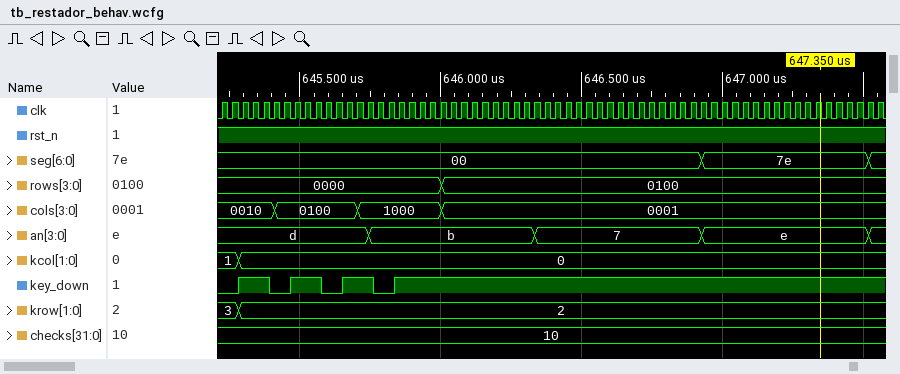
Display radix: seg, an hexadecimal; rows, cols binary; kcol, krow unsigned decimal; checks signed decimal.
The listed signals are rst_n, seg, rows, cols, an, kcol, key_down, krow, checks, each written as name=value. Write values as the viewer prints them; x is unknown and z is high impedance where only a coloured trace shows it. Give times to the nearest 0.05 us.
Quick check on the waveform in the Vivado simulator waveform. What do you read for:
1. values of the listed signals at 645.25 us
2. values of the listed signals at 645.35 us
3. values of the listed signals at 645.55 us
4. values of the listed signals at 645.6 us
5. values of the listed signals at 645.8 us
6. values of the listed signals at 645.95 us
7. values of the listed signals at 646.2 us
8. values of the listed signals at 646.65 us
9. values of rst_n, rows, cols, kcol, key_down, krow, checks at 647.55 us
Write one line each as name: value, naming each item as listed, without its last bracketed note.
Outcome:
values of the listed signals at 645.25 us: rst_n=1, seg=00, rows=0000, cols=0010, an=d, kcol=1, key_down=0, krow=3, checks=10
values of the listed signals at 645.35 us: rst_n=1, seg=00, rows=0000, cols=0010, an=d, kcol=0, key_down=1, krow=2, checks=10
values of the listed signals at 645.55 us: rst_n=1, seg=00, rows=0000, cols=0100, an=d, kcol=0, key_down=1, krow=2, checks=10
values of the listed signals at 645.6 us: rst_n=1, seg=00, rows=0000, cols=0100, an=d, kcol=0, key_down=0, krow=2, checks=10
values of the listed signals at 645.8 us: rst_n=1, seg=00, rows=0000, cols=1000, an=b, kcol=0, key_down=0, krow=2, checks=10
values of the listed signals at 645.95 us: rst_n=1, seg=00, rows=0000, cols=1000, an=b, kcol=0, key_down=1, krow=2, checks=10
values of the listed signals at 646.2 us: rst_n=1, seg=00, rows=0100, cols=0001, an=b, kcol=0, key_down=1, krow=2, checks=10
values of the listed signals at 646.65 us: rst_n=1, seg=00, rows=0100, cols=0001, an=7, kcol=0, key_down=1, krow=2, checks=10
values of rst_n, rows, cols, kcol, key_down, krow, checks at 647.55 us: rst_n=1, rows=0100, cols=0001, kcol=0, key_down=1, krow=2, checks=10
